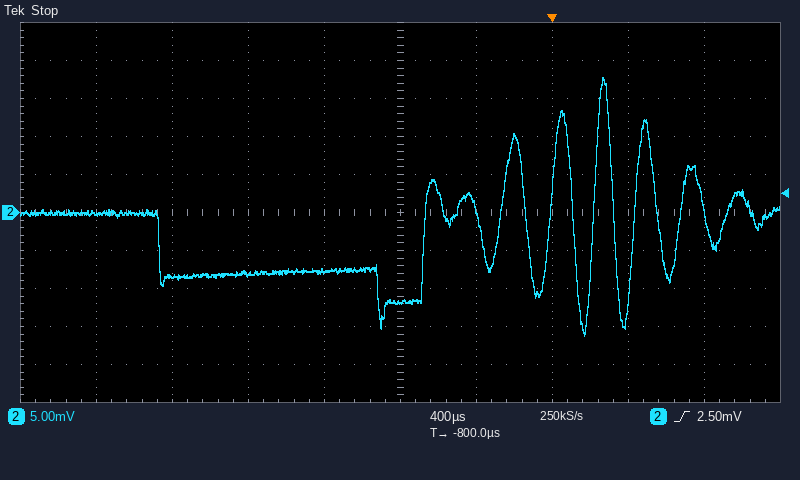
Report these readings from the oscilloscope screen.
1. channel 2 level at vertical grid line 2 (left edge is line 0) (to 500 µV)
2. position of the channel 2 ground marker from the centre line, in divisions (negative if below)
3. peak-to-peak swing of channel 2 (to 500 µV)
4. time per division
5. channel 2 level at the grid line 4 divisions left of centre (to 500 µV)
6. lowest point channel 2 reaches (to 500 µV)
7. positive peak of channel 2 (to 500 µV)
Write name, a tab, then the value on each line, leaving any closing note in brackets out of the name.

channel 2 level at vertical grid line 2 (left edge is line 0)	-8.5 mV
position of the channel 2 ground marker from the centre line, in divisions	0.0 div
peak-to-peak swing of channel 2	34.0 mV
time per division	400 µs
channel 2 level at the grid line 4 divisions left of centre	0.0 mV
lowest point channel 2 reaches	-16.0 mV
positive peak of channel 2	18.0 mV
